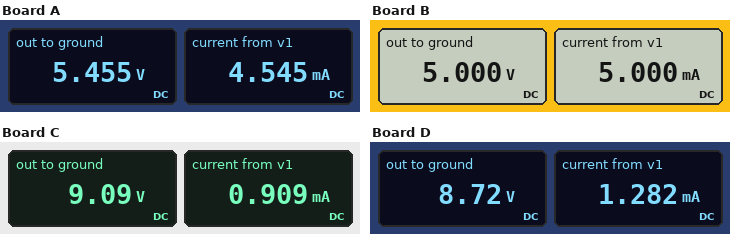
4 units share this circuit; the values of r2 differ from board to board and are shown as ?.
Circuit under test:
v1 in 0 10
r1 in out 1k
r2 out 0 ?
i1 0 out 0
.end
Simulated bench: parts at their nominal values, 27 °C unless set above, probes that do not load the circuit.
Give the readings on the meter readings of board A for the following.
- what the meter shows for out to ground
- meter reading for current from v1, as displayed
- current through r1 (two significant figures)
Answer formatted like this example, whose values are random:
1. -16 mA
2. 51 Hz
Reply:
1. 5.455 V
2. 4.545 mA
3. 4.5 mA
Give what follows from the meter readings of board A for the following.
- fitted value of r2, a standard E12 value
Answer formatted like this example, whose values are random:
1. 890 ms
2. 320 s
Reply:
1. 1.2 kΩ
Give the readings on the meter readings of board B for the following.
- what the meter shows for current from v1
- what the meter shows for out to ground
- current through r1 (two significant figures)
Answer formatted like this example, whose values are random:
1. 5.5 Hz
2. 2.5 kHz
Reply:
1. 5.000 mA
2. 5.000 V
3. 5.0 mA
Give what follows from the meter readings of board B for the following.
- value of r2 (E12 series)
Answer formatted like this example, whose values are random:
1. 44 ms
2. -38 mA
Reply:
1. 1 kΩ
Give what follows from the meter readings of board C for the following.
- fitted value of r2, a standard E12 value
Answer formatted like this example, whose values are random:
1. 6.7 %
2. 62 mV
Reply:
1. 10 kΩ
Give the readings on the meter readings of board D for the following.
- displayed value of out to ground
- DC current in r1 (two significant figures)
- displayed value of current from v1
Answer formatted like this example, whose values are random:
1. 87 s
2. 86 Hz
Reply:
1. 8.72 V
2. 1.3 mA
3. 1.282 mA
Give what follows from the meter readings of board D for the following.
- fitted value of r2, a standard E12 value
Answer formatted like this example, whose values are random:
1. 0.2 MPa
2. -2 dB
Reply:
1. 6.8 kΩ
